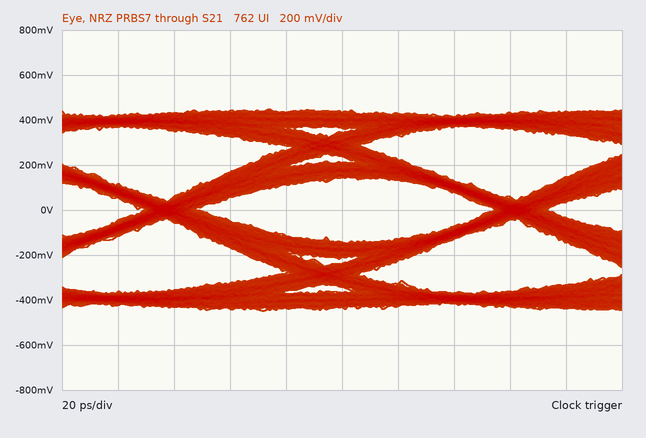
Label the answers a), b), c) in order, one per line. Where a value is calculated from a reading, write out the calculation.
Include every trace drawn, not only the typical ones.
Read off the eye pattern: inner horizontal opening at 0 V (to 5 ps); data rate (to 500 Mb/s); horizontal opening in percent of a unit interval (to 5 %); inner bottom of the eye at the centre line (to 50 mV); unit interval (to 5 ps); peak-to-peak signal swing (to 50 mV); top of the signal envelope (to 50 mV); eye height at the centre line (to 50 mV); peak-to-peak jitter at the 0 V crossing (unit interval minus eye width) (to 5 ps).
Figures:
a) 105 ps
b) 8.0 Gb/s
c) 105 ps / 125 ps ≈ 84.0 %, so 85 % to the nearest 5 %
d) -150 mV
e) 125 ps
f) 900 mV
g) 450 mV
h) 300 mV
i) 20 ps
